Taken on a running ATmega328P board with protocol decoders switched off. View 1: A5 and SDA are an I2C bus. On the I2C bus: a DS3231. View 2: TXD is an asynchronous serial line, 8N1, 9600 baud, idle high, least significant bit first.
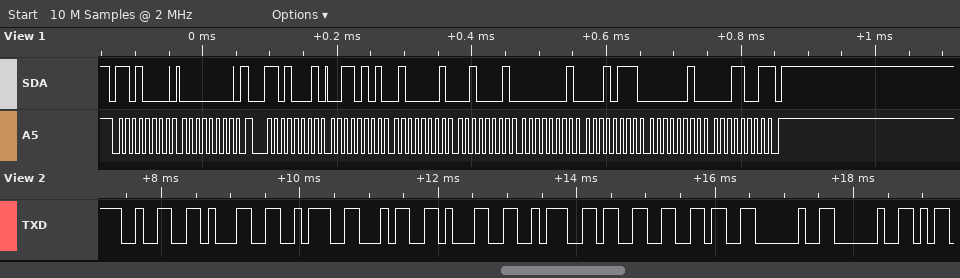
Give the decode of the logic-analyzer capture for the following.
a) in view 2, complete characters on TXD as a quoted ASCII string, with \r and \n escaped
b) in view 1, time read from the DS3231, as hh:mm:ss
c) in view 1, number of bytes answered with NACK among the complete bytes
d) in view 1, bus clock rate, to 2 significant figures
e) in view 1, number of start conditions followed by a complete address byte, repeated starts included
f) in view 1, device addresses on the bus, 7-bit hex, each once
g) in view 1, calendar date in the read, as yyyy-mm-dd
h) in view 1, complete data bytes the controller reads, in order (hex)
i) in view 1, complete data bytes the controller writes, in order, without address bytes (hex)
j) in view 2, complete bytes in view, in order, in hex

"21:41:36  "
21:41:35
1
100 kHz
2
0x68
2019-02-17
35 41 21 01 17 02 19
00
0x32 0x31 0x3A 0x34 0x31 0x3A 0x33 0x36 0x20 0x20
